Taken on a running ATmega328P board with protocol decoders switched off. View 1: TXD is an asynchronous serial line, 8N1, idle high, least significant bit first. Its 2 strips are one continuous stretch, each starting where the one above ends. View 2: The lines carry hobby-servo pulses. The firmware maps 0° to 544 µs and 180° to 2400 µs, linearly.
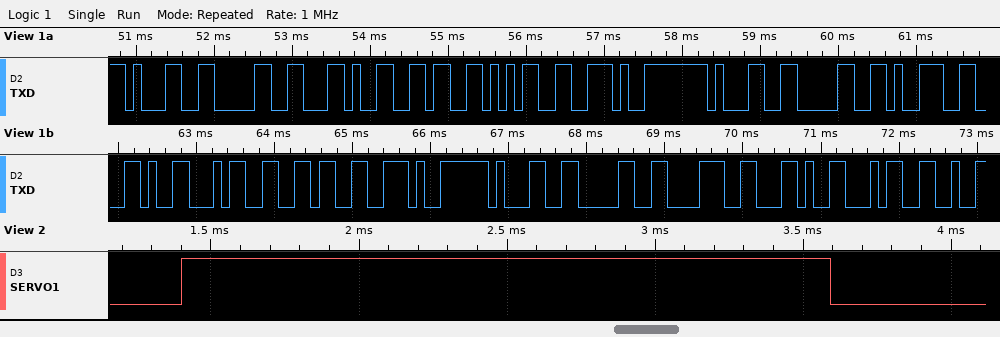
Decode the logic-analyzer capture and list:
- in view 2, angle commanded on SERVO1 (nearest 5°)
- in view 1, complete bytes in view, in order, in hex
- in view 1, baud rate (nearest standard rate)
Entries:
160°
31 30 2C 36 35 2E 31 30 39 2C 34 36 2E 31 30 38 2C 34
9600 baud
